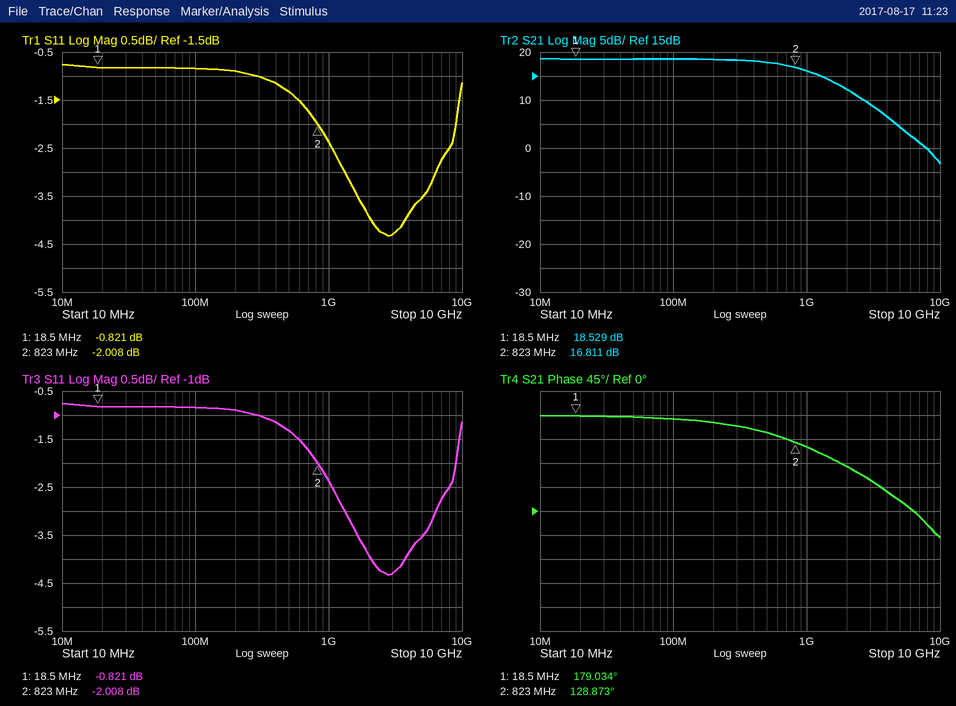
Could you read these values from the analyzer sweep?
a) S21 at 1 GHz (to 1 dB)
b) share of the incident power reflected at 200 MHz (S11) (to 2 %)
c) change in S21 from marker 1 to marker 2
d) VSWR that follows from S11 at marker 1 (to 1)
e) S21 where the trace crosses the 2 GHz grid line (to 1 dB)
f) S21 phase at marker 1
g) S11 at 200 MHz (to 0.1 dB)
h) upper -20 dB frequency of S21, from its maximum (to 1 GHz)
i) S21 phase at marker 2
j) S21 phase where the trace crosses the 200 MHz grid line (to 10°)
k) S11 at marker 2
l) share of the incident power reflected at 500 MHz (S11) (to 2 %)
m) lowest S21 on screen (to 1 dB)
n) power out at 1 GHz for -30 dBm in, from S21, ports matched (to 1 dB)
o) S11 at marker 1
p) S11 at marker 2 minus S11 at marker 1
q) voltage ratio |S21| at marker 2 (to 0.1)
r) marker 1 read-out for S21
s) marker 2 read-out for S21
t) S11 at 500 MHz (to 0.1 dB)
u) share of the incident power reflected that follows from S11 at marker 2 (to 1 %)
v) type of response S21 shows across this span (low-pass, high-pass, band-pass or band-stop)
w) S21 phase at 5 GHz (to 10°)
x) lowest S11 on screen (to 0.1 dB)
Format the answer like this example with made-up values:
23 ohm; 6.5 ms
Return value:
16 dB; 82 %; -1.718 dB; 21; 12 dB; 179.034°; -0.9 dB; 9 GHz; 128.873°; 170°; -2.008 dB; 74 %; -3 dB; -14 dBm; -0.821 dB; -1.187 dB; 6.9; 18.529 dB; 16.811 dB; -1.3 dB; 63 %; low-pass; 20°; -4.3 dB
